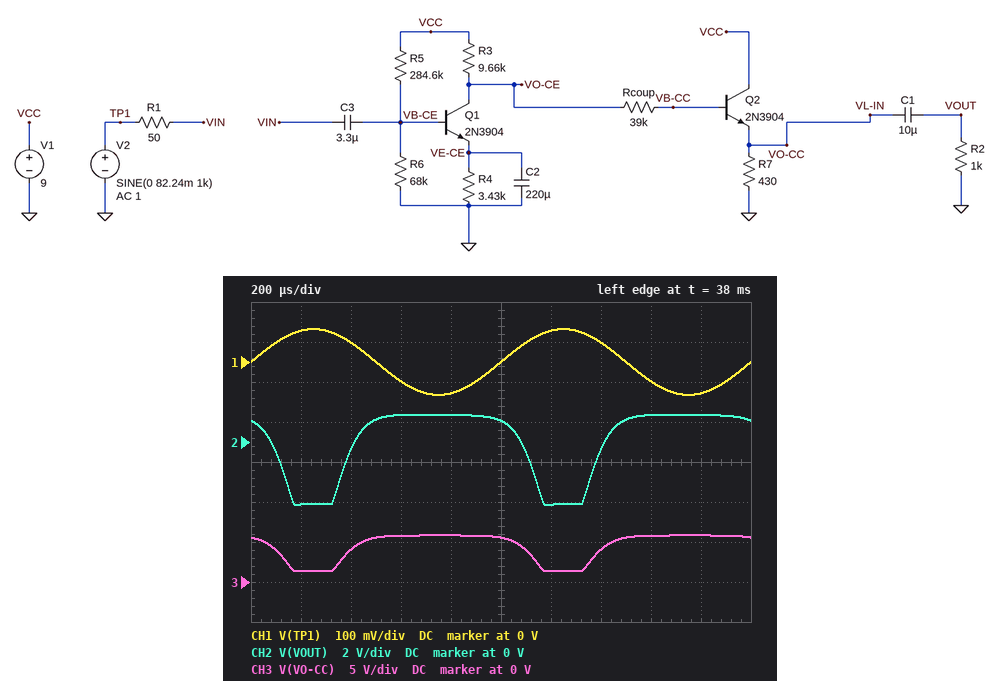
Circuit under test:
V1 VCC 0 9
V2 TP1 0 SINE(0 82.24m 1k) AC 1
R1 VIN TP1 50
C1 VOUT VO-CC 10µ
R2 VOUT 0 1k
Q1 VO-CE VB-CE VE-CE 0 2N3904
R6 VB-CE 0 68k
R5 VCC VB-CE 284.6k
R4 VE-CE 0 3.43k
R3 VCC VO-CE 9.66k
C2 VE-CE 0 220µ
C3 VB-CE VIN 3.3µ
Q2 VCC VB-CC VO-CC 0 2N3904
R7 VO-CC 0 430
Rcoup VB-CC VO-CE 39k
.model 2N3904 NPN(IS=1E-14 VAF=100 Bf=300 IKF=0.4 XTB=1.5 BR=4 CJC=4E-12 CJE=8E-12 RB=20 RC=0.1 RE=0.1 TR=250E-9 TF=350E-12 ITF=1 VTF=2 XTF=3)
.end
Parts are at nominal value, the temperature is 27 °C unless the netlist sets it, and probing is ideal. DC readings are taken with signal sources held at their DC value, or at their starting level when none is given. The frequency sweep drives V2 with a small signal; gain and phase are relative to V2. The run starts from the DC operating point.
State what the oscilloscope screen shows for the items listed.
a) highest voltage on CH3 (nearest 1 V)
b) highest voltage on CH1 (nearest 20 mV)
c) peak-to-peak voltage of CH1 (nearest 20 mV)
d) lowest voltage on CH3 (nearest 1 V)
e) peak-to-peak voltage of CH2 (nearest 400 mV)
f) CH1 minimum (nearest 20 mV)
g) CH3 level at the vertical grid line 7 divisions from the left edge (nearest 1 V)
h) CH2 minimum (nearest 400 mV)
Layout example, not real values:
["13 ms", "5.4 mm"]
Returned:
["6 V", "80 mV", "160 mV", "1 V", "4.4 V", "-80 mV", "4 V", "-3.2 V"]
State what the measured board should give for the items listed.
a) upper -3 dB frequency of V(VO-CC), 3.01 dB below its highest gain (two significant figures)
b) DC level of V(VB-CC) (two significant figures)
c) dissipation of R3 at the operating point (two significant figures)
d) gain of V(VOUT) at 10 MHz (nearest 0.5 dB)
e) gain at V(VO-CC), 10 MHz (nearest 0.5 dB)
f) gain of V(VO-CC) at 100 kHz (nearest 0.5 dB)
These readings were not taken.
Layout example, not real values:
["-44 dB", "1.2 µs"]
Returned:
["1.3 MHz", "4.6 V", "1.1 mW", "13.5 dB", "13.5 dB", "37.0 dB"]
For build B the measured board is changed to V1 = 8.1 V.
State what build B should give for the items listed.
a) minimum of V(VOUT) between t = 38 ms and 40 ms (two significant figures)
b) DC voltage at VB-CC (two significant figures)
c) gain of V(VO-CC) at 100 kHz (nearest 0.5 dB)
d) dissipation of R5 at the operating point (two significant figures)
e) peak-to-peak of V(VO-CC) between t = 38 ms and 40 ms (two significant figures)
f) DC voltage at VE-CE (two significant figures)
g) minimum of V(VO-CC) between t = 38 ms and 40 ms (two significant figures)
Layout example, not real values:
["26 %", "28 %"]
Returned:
["-2.8 V", "4.3 V", "35.5 dB", "150 µW", "4.0 V", "900 mV", "1.2 V"]
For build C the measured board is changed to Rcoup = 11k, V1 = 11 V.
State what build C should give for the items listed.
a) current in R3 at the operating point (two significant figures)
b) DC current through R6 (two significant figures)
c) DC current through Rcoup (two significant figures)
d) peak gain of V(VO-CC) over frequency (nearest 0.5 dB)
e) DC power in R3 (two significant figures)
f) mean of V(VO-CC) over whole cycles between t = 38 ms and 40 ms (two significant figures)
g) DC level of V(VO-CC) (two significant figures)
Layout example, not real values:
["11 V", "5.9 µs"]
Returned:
["450 µA", "30 µA", "41 µA", "41.5 dB", "2.0 mW", "6.6 V", "5.4 V"]
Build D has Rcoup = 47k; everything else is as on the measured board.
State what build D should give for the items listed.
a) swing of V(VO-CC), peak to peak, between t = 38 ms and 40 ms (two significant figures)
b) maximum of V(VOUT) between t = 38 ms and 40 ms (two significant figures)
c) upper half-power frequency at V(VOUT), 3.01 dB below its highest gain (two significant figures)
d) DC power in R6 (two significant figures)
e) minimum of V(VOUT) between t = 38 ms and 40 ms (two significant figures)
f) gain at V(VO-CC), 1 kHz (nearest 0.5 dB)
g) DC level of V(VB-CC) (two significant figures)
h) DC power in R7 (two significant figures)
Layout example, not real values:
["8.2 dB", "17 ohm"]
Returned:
["4.3 V", "1.3 V", "1.2 MHz", "42 µW", "-3.0 V", "36.5 dB", "4.4 V", "32 mW"]
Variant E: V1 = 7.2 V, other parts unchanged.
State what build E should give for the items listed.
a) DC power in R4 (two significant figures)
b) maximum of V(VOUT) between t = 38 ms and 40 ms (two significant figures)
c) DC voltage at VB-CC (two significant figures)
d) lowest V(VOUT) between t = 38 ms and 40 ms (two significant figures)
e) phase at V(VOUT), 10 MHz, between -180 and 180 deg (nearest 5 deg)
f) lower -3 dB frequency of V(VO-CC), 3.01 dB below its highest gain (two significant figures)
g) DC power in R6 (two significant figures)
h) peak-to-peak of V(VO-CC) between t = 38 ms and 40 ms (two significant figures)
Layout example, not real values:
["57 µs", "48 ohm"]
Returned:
["160 µW", "1.1 V", "3.9 V", "-2.5 V", "35 deg", "6.4 Hz", "27 µW", "3.5 V"]
